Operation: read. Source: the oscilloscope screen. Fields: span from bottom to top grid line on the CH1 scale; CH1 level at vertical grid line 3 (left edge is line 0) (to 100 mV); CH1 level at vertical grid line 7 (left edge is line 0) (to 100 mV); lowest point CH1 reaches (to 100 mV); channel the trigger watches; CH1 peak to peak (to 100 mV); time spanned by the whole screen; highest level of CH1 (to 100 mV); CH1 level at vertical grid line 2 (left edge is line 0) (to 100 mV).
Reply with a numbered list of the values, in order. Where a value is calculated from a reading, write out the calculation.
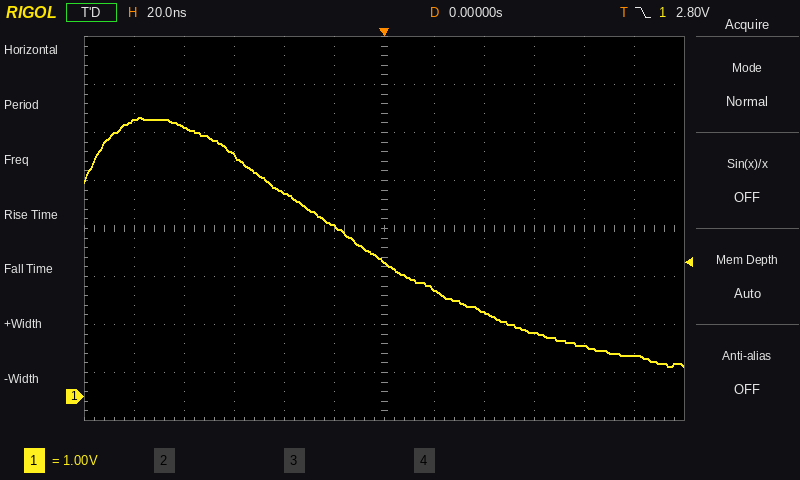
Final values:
1. 8 V
2. 5.0 V
3. 2.2 V
4. 600 mV
5. CH1
6. 5.8 V − (600 mV) = 5.2 V
7. 240 ns
8. 5.8 V
9. 5.6 V
